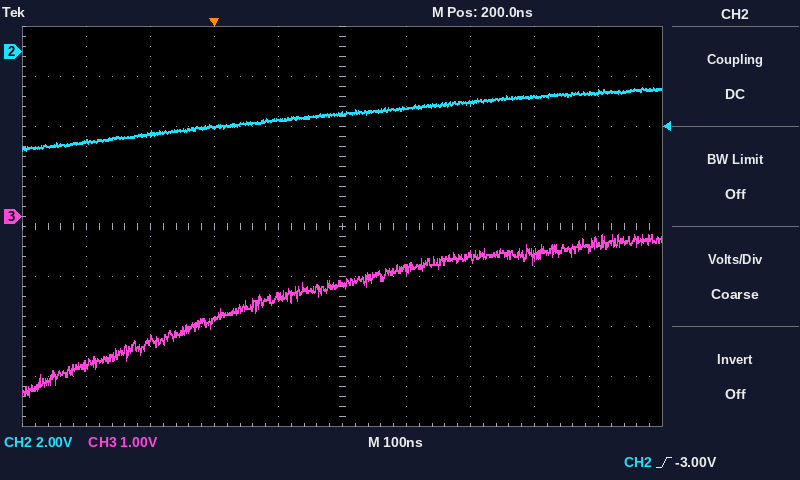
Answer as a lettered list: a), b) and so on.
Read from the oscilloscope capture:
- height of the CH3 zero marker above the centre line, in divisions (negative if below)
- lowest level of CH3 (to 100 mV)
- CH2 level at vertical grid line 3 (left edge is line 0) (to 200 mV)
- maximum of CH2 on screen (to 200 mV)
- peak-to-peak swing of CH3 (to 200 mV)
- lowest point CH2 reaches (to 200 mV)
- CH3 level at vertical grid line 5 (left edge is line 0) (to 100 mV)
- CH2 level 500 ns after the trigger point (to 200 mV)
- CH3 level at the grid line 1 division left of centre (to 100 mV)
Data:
a) +0.2 div
b) -3.6 V
c) -3.0 V
d) -1.4 V
e) 3.2 V
f) -4.0 V
g) -1.3 V
h) -1.8 V
i) -1.6 V
